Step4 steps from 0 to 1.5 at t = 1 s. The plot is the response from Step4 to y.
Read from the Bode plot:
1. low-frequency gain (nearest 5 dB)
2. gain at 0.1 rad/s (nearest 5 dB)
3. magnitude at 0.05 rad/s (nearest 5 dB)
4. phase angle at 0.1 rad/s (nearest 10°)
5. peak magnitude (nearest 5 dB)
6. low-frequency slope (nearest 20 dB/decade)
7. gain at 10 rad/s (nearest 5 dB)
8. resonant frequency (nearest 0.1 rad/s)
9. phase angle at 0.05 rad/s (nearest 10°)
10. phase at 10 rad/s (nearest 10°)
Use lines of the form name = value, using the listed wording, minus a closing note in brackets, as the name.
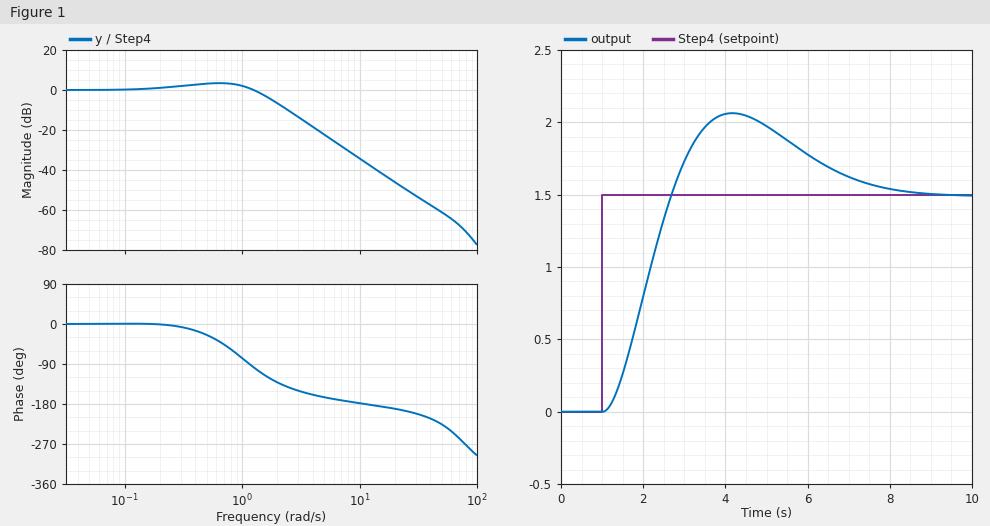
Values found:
low-frequency gain = 0 dB
gain at 0.1 rad/s = 0 dB
magnitude at 0.05 rad/s = 0 dB
phase angle at 0.1 rad/s = 0°
peak magnitude = 5 dB
low-frequency slope = 0 dB/decade
gain at 10 rad/s = -35 dB
resonant frequency = 0.6 rad/s
phase angle at 0.05 rad/s = 0°
phase at 10 rad/s = -180°
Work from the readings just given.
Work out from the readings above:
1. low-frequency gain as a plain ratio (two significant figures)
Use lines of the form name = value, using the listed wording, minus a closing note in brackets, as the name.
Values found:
low-frequency gain as a plain ratio = 1.0
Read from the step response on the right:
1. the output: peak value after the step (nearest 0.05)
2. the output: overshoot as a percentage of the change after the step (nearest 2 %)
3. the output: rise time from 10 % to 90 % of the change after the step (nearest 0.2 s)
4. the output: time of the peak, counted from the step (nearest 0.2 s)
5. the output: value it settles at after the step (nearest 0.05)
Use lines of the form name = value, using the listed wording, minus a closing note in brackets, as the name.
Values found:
the output: peak value after the step = 2.05
the output: overshoot as a percentage of the change after the step = 38 %
the output: rise time from 10 % to 90 % of the change after the step = 1.2 s
the output: time of the peak, counted from the step = 3.2 s
the output: value it settles at after the step = 1.50
